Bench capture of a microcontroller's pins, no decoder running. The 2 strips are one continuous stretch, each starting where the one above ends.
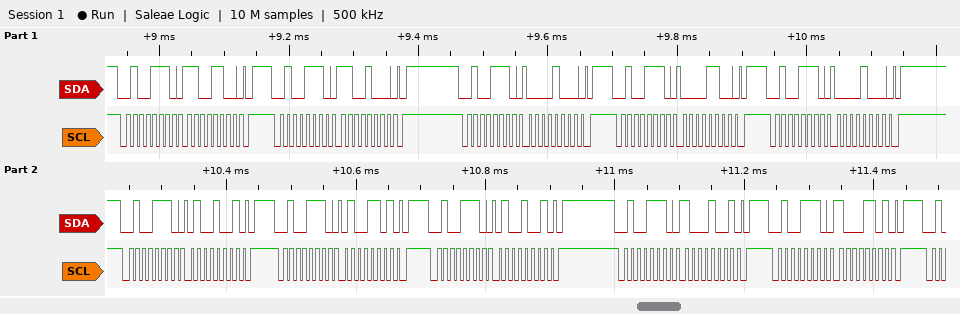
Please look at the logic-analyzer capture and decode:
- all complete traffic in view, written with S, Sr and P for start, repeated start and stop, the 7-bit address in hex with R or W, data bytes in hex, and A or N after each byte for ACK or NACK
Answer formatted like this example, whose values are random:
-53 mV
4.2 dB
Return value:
S 27W A CC A P S 27W A C8 A P S 27W A 08 A P S 27W A 0C A P S 27W A 08 A P S 27W A 49 A P S 27W A 4D A P S 27W A 49 A P S 27W A 89 A P S 27W A 8D A P
